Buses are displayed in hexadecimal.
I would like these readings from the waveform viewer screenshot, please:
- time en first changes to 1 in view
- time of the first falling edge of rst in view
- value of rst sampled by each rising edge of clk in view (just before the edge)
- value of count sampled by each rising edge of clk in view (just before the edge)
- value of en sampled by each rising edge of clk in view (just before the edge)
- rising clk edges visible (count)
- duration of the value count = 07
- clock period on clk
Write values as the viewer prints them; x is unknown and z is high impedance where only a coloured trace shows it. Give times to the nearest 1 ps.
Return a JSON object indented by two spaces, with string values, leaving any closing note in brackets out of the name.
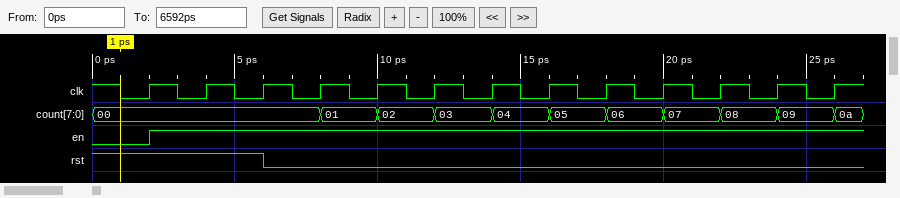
{
  "time en first changes to 1 in view": "2 ps",
  "time of the first falling edge of rst in view": "6 ps",
  "value of rst sampled by each rising edge of clk in view": "1 1 1 0 0 0 0 0 0 0 0 0 0",
  "value of count sampled by each rising edge of clk in view": "00, 00, 00, 00, 01, 02, 03, 04, 05, 06, 07, 08, 09",
  "value of en sampled by each rising edge of clk in view": "0 1 1 1 1 1 1 1 1 1 1 1 1",
  "rising clk edges visible": "13",
  "duration of the value count = 07": "2 ps",
  "clock period on clk": "2 ps"
}
